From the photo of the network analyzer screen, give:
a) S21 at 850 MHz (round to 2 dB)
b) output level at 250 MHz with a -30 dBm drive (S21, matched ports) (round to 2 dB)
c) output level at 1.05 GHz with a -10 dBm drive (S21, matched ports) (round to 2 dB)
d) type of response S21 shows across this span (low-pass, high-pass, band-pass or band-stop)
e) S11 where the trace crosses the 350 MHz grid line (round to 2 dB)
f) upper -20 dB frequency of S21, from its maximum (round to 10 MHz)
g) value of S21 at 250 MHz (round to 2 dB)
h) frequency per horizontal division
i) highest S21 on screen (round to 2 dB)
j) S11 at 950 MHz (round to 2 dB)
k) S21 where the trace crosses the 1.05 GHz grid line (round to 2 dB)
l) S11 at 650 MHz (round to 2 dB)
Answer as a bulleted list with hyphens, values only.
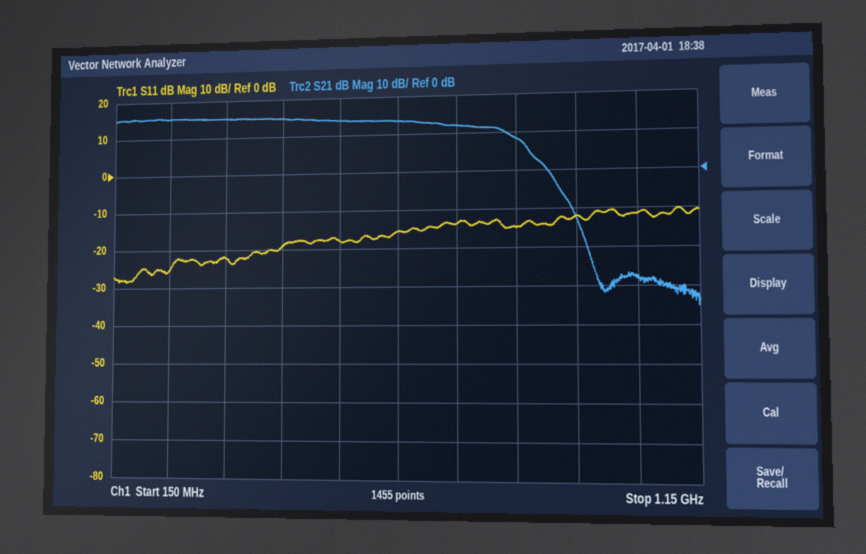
- 8 dB
- -14 dBm
- -38 dBm
- low-pass
- -22 dB
- 920 MHz
- 16 dB
- 100 MHz
- 16 dB
- -12 dB
- -28 dB
- -16 dB
